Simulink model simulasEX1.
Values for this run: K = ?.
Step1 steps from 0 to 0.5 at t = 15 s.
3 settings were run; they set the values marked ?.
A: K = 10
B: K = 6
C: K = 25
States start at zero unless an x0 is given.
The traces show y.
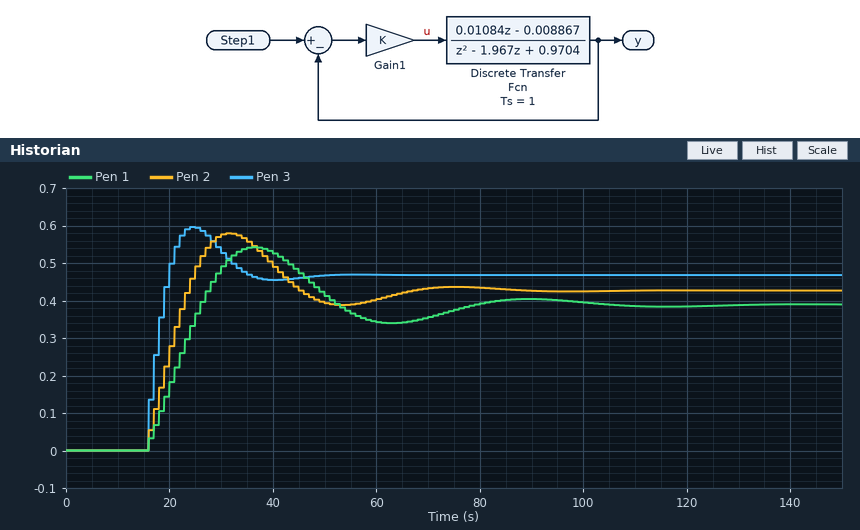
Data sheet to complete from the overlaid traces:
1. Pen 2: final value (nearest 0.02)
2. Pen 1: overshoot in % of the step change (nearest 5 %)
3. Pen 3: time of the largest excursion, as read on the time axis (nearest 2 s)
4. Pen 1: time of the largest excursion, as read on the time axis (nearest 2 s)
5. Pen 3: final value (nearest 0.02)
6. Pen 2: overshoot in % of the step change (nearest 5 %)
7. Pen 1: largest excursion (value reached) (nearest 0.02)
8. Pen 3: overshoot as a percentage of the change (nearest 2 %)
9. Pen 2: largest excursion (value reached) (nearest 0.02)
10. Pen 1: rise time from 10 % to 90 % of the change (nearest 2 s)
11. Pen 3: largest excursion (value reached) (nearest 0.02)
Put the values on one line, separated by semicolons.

0.42; 40 %; 24 s; 36 s; 0.46; 35 %; 0.54; 28 %; 0.58; 8 s; 0.60
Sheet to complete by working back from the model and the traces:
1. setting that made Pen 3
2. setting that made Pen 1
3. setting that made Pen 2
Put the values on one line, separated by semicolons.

C; B; A
